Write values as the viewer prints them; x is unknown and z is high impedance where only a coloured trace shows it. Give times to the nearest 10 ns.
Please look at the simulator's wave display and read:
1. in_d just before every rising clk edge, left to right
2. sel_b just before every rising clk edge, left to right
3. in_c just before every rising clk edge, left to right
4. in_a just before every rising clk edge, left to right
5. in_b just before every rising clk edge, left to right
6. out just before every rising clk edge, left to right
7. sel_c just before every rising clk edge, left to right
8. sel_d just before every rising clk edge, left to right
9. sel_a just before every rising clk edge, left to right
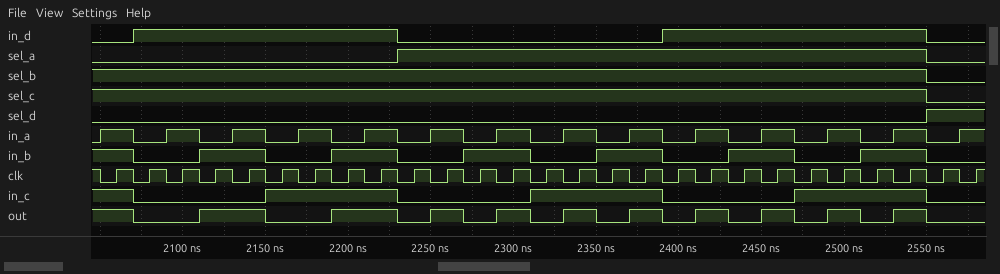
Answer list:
0 1 1 1 1 1 1 1 1 0 0 0 0 0 0 0 0 1 1 1 1 1 1 1 1 0 0
1 1 1 1 1 1 1 1 1 1 1 1 1 1 1 1 1 1 1 1 1 1 1 1 1 0 0
1 0 0 0 0 1 1 1 1 0 0 0 0 1 1 1 1 0 0 0 0 1 1 1 1 0 0
1 0 1 0 1 0 1 0 1 0 1 0 1 0 1 0 1 0 1 0 1 0 1 0 1 0 1
1 0 0 1 1 0 0 1 1 0 0 1 1 0 0 1 1 0 0 1 1 0 0 1 1 0 0
1 0 0 1 1 0 0 1 1 0 1 0 1 0 1 0 1 0 1 0 1 0 1 0 1 0 0
1 1 1 1 1 1 1 1 1 1 1 1 1 1 1 1 1 1 1 1 1 1 1 1 1 0 0
0 0 0 0 0 0 0 0 0 0 0 0 0 0 0 0 0 0 0 0 0 0 0 0 0 1 1
0 0 0 0 0 0 0 0 0 1 1 1 1 1 1 1 1 1 1 1 1 1 1 1 1 0 0
